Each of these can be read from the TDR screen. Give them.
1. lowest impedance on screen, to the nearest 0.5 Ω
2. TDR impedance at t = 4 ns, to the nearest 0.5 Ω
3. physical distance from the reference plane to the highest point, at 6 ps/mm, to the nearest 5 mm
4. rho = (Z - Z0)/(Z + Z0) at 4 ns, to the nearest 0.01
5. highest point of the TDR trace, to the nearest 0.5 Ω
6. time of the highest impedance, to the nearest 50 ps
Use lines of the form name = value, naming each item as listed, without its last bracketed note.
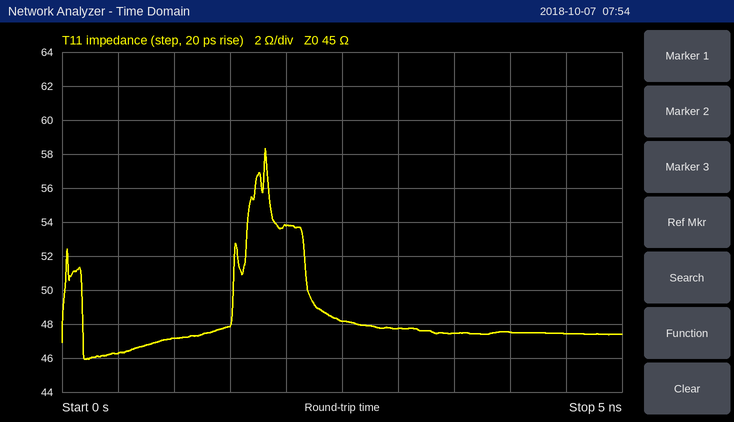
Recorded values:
lowest impedance on screen, to the nearest 0.5 Ω = 46.0 Ω
TDR impedance at t = 4 ns, to the nearest 0.5 Ω = 47.5 Ω
physical distance from the reference plane to the highest point, at 6 ps/mm, to the nearest 5 mm = 150 mm
rho = (Z - Z0)/(Z + Z0) at 4 ns, to the nearest 0.01 = +0.03
highest point of the TDR trace, to the nearest 0.5 Ω = 58.5 Ω
time of the highest impedance, to the nearest 50 ps = 1.80 ns
